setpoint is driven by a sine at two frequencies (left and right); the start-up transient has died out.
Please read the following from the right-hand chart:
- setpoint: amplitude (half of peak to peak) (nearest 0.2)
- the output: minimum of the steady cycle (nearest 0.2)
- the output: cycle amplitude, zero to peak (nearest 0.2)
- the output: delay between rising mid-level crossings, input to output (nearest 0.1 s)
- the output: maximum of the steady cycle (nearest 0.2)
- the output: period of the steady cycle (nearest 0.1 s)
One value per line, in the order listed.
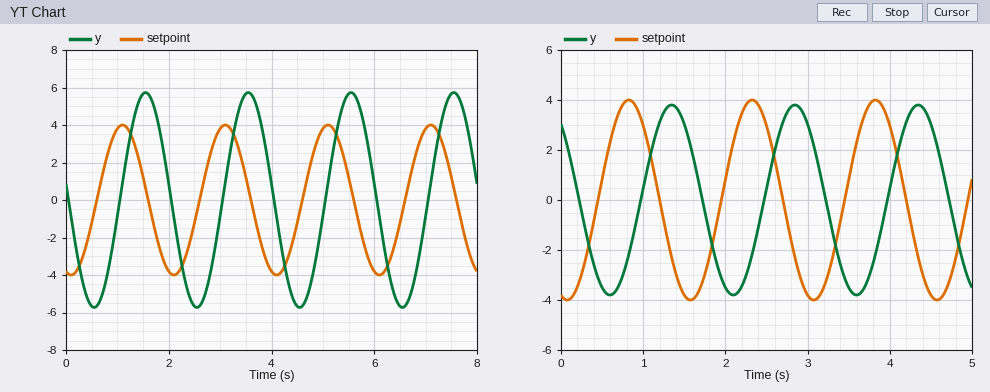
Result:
4.0
-3.8
3.8
0.5 s
3.8
1.5 s
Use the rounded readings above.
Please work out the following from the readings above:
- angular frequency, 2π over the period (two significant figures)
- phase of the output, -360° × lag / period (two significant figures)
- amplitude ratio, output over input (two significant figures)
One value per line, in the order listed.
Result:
4.2 rad/s
-120°
0.95
